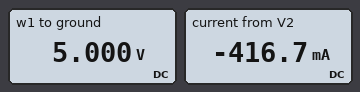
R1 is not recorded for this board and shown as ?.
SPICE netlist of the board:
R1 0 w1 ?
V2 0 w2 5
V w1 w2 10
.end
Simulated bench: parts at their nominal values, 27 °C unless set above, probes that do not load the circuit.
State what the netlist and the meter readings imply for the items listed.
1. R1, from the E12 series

12 Ω
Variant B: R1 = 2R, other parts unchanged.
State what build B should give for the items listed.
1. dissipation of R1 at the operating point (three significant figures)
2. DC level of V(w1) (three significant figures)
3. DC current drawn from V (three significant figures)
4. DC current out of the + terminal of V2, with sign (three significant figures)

12.5 W
5.00 V
2.50 A
-2.50 A
